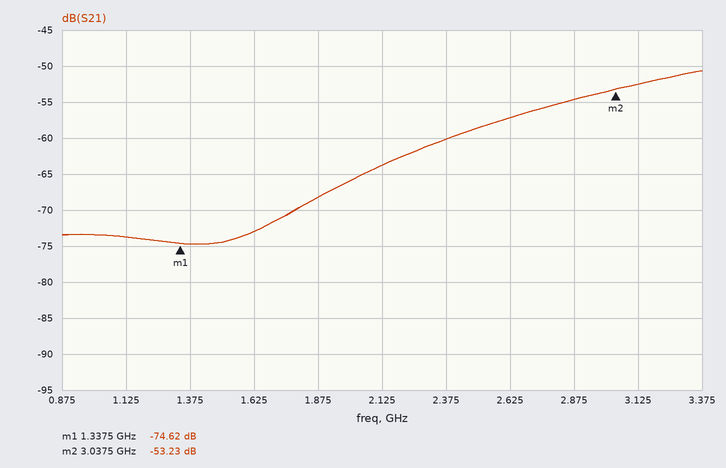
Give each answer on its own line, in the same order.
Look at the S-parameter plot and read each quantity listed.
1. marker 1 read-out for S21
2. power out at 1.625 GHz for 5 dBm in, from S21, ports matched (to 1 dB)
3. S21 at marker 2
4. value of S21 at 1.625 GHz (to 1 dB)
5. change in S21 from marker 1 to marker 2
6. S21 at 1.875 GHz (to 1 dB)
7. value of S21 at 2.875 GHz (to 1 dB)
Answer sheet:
-74.62 dB
-68 dBm
-53.23 dB
-73 dB
21.39 dB
-68 dB
-55 dB
